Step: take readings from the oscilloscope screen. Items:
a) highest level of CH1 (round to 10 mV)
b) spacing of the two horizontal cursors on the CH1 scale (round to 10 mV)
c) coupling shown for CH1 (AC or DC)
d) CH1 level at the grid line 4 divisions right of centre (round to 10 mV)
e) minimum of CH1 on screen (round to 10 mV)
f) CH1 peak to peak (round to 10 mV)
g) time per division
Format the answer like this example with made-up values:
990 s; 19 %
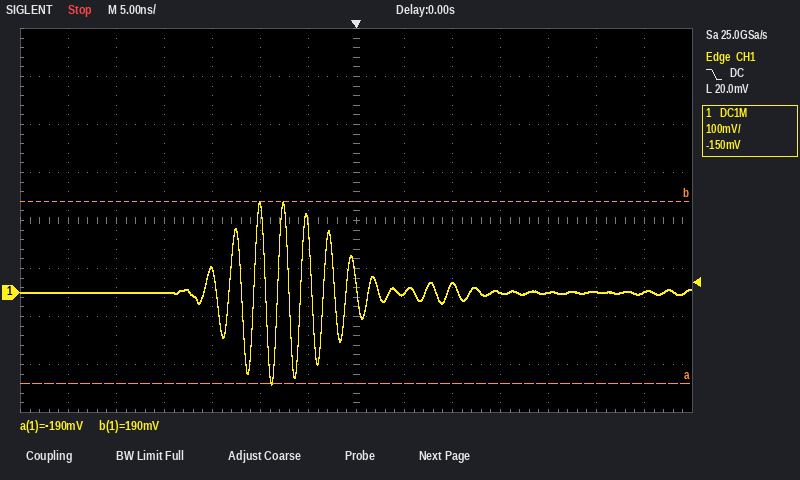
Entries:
190 mV; 380 mV; DC; 0 mV; -190 mV; 380 mV; 5 ns
